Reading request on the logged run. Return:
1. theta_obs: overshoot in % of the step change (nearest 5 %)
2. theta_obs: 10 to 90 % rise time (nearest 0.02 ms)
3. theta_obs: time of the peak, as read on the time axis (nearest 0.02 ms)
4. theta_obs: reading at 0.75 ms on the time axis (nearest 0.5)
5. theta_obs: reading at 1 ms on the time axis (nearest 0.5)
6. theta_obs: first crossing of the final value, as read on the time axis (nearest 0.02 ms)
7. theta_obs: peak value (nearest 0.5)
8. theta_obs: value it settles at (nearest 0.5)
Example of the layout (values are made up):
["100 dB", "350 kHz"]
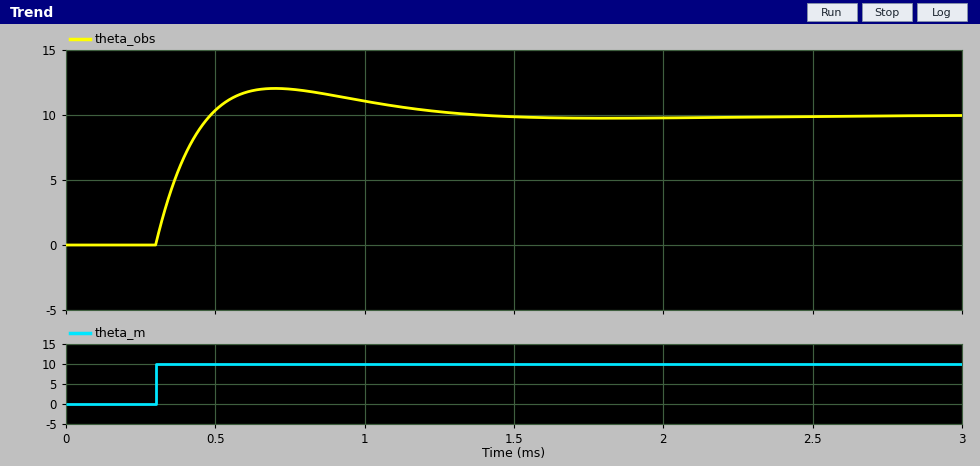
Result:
["20 %", "0.14 ms", "0.70 ms", "12.0", "11.0", "0.48 ms", "12.0", "10.0"]
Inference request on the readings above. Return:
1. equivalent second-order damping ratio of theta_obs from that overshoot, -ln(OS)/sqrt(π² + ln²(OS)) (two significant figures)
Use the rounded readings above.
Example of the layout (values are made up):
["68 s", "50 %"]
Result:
["0.46"]
